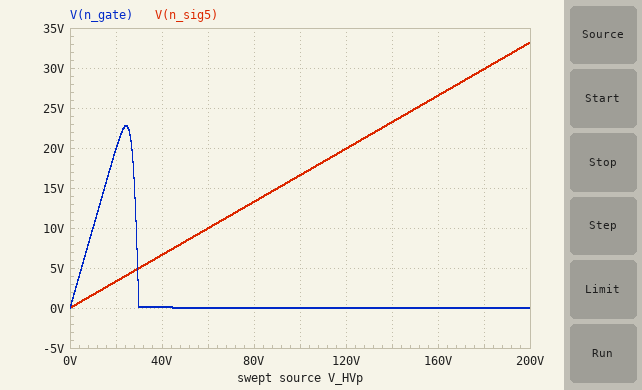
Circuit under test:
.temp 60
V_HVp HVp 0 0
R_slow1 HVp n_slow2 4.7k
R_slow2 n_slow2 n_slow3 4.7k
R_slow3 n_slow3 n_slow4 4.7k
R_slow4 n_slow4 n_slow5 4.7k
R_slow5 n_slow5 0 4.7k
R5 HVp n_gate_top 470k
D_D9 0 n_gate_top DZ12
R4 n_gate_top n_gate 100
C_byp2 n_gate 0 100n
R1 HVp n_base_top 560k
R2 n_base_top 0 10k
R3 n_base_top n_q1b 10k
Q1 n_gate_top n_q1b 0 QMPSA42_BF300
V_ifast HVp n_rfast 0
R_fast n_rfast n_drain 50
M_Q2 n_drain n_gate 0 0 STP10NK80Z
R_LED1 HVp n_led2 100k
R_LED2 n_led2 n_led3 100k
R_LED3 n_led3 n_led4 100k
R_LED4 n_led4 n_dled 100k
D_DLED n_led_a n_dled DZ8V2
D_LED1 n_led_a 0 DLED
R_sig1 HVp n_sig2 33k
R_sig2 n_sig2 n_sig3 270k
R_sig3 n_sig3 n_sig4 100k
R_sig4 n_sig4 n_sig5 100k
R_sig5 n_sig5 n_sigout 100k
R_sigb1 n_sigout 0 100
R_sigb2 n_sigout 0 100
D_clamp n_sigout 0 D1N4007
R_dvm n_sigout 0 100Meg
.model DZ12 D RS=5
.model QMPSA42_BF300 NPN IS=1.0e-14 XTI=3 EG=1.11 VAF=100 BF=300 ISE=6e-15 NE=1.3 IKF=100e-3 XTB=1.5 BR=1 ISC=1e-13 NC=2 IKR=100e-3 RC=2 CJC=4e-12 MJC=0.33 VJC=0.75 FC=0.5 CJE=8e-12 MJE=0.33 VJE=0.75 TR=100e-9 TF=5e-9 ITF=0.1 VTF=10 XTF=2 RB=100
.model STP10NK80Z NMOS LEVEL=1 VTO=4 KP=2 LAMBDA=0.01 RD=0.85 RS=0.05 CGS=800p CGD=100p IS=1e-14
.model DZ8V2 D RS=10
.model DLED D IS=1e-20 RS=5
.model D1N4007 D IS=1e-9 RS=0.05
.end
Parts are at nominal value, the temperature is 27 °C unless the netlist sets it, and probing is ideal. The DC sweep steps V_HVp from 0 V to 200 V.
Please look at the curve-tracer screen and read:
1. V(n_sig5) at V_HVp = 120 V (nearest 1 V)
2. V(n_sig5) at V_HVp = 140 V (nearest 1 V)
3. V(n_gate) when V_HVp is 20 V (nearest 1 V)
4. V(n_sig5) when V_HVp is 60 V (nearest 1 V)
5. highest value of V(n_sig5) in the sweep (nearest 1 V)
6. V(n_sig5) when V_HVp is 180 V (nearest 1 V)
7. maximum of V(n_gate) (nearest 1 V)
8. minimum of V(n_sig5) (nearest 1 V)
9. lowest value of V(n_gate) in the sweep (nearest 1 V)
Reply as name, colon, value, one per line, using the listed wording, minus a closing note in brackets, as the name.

V(n_sig5) at V_HVp = 120 V: 20 V
V(n_sig5) at V_HVp = 140 V: 23 V
V(n_gate) when V_HVp is 20 V: 20 V
V(n_sig5) when V_HVp is 60 V: 10 V
highest value of V(n_sig5) in the sweep: 33 V
V(n_sig5) when V_HVp is 180 V: 30 V
maximum of V(n_gate): 23 V
minimum of V(n_sig5): 0 V
lowest value of V(n_gate) in the sweep: 0 V
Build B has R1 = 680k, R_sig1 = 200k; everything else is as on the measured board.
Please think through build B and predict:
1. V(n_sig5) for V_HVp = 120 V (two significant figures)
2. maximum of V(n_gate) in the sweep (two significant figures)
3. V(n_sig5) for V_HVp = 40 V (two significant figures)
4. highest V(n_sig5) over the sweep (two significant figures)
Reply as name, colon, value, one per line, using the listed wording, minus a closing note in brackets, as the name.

V(n_sig5) for V_HVp = 120 V: 16 V
maximum of V(n_gate) in the sweep: 28 V
V(n_sig5) for V_HVp = 40 V: 5.2 V
highest V(n_sig5) over the sweep: 26 V
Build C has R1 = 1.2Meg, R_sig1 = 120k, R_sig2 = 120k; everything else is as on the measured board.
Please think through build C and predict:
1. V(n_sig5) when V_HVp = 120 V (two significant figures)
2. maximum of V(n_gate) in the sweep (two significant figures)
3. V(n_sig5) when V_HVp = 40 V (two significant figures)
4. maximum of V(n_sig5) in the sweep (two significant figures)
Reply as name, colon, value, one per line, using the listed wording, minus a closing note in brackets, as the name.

V(n_sig5) when V_HVp = 120 V: 22 V
maximum of V(n_gate) in the sweep: 50 V
V(n_sig5) when V_HVp = 40 V: 7.4 V
maximum of V(n_sig5) in the sweep: 37 V
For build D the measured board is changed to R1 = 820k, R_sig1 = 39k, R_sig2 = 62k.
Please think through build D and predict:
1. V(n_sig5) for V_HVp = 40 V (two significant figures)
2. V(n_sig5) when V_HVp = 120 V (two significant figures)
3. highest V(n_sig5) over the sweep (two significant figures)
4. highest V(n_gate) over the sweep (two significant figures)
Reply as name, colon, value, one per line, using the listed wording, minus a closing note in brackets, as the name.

V(n_sig5) for V_HVp = 40 V: 10 V
V(n_sig5) when V_HVp = 120 V: 30 V
highest V(n_sig5) over the sweep: 50 V
highest V(n_gate) over the sweep: 34 V
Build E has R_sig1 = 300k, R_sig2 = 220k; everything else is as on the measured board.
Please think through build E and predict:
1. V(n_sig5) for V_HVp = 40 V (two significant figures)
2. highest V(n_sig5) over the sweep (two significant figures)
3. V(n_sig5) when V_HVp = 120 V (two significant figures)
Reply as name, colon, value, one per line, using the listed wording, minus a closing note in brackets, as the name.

V(n_sig5) for V_HVp = 40 V: 4.9 V
highest V(n_sig5) over the sweep: 24 V
V(n_sig5) when V_HVp = 120 V: 15 V
